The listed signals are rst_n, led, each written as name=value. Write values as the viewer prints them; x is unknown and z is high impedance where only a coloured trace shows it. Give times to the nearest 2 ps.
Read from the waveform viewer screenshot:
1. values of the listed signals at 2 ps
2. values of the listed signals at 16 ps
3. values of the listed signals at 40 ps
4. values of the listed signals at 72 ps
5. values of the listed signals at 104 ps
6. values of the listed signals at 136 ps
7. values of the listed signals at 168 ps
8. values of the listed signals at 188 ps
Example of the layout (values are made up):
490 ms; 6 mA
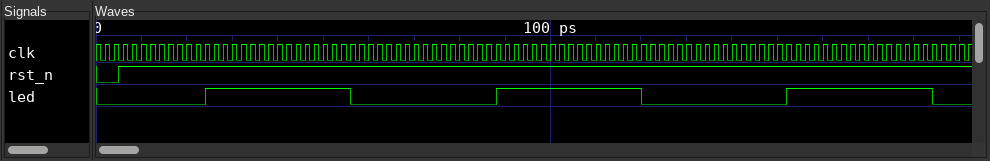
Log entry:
rst_n=0, led=0; rst_n=1, led=0; rst_n=1, led=1; rst_n=1, led=0; rst_n=1, led=1; rst_n=1, led=0; rst_n=1, led=1; rst_n=1, led=0
